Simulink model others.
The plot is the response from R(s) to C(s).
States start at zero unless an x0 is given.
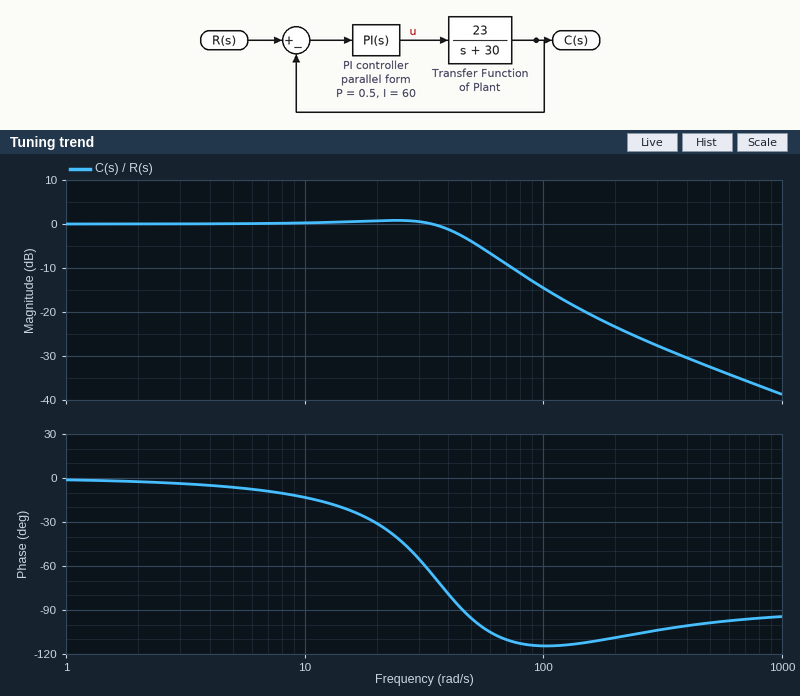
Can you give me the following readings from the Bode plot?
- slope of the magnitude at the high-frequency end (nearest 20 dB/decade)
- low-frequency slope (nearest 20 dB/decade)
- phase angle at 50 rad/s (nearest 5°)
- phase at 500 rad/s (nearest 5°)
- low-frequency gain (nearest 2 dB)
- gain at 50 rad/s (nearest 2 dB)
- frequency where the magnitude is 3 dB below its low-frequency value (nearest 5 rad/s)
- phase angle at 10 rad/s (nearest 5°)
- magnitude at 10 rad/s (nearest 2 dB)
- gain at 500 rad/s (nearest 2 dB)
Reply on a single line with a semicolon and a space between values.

-20 dB/decade; 0 dB/decade; -95°; -100°; 0 dB; -4 dB; 45 rad/s; -15°; 0 dB; -32 dB
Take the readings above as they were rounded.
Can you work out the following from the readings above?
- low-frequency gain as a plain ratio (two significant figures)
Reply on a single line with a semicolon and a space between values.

1.0
